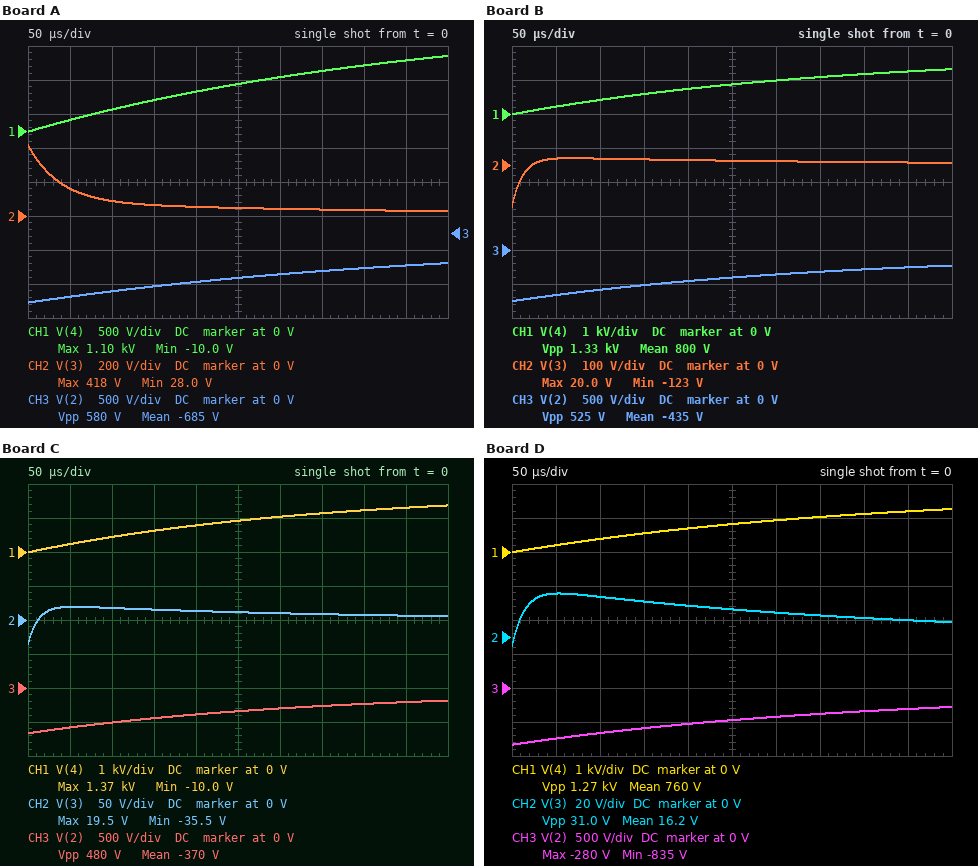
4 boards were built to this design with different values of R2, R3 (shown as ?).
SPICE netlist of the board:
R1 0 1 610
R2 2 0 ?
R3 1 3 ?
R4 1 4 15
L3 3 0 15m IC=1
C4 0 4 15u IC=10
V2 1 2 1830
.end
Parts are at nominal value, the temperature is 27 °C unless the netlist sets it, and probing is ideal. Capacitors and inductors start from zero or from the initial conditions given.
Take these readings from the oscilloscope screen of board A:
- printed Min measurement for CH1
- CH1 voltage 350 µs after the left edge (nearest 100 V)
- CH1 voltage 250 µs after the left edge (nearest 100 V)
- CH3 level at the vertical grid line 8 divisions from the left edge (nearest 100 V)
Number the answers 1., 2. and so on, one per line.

1. -10.0 V
2. 900 V
3. 700 V
4. -500 V
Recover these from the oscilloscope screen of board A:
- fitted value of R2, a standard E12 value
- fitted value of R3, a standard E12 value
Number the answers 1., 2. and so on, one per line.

1. 18 Ω
2. 390 Ω
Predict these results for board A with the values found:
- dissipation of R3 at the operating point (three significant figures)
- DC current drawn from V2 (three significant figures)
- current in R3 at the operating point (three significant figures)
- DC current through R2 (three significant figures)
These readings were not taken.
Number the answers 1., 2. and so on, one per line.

1. 7.42 kW
2. 7.15 A
3. 4.36 A
4. 7.15 A
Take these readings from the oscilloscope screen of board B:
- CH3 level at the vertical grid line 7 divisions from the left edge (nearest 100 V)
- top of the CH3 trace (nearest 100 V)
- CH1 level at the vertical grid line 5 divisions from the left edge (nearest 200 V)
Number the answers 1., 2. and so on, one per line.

1. -300 V
2. -200 V
3. 800 V
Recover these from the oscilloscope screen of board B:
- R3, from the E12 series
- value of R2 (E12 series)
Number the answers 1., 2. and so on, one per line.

1. 1.2 kΩ
2. 10 Ω
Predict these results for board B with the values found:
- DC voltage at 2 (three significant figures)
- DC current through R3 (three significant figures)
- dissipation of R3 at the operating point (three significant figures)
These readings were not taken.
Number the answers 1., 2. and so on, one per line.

1. -44.2 V
2. 1.49 A
3. 2.66 kW
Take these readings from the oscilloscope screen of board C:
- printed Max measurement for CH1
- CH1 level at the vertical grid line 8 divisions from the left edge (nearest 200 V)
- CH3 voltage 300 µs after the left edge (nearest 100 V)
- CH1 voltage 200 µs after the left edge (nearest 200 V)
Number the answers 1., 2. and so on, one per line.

1. 1.37 kV
2. 1.2 kV
3. -300 V
4. 800 V
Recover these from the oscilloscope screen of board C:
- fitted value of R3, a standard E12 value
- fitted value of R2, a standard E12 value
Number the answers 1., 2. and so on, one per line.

1. 1.2 kΩ
2. 8.2 Ω
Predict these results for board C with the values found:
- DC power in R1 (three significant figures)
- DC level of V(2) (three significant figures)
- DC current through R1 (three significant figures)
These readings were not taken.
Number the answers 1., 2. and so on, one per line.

1. 5.27 kW
2. -36.4 V
3. 2.94 A
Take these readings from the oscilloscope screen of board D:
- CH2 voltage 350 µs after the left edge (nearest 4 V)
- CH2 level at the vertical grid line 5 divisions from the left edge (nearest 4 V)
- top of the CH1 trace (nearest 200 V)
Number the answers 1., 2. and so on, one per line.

1. 12 V
2. 16 V
3. 1.2 kV
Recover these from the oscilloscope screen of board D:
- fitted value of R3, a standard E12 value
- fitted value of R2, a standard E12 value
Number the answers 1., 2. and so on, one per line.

1. 1 kΩ
2. 12 Ω
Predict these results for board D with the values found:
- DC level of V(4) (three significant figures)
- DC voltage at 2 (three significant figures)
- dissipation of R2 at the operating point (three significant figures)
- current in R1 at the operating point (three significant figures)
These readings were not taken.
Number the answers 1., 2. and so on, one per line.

1. 1.77 kV
2. -56.2 V
3. 263 W
4. 2.91 A
